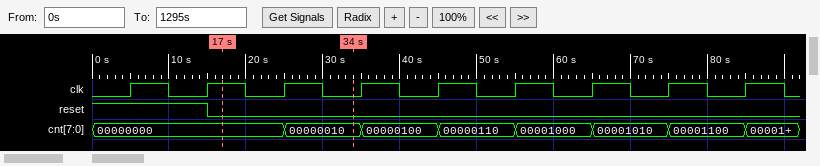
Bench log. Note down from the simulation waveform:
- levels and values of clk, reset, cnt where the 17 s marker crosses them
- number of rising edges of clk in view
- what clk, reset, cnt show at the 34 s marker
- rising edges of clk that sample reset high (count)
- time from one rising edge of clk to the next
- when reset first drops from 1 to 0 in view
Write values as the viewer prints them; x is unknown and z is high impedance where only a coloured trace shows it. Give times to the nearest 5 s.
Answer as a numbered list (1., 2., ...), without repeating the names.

1. clk=1, reset=0, cnt=00000000
2. 9
3. clk=0, reset=0, cnt=00000010
4. 2
5. 10 s
6. 15 s
